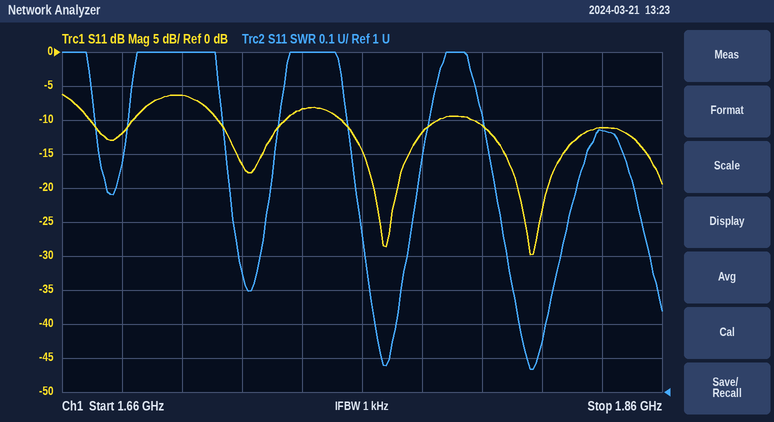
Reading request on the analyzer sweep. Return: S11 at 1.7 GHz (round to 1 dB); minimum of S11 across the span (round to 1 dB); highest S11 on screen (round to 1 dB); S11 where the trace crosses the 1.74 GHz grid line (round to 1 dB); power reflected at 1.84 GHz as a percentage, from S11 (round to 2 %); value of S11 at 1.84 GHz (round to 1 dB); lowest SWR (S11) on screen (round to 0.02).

-6 dB
-30 dB
-6 dB
-8 dB
8 %
-11 dB
1.06
